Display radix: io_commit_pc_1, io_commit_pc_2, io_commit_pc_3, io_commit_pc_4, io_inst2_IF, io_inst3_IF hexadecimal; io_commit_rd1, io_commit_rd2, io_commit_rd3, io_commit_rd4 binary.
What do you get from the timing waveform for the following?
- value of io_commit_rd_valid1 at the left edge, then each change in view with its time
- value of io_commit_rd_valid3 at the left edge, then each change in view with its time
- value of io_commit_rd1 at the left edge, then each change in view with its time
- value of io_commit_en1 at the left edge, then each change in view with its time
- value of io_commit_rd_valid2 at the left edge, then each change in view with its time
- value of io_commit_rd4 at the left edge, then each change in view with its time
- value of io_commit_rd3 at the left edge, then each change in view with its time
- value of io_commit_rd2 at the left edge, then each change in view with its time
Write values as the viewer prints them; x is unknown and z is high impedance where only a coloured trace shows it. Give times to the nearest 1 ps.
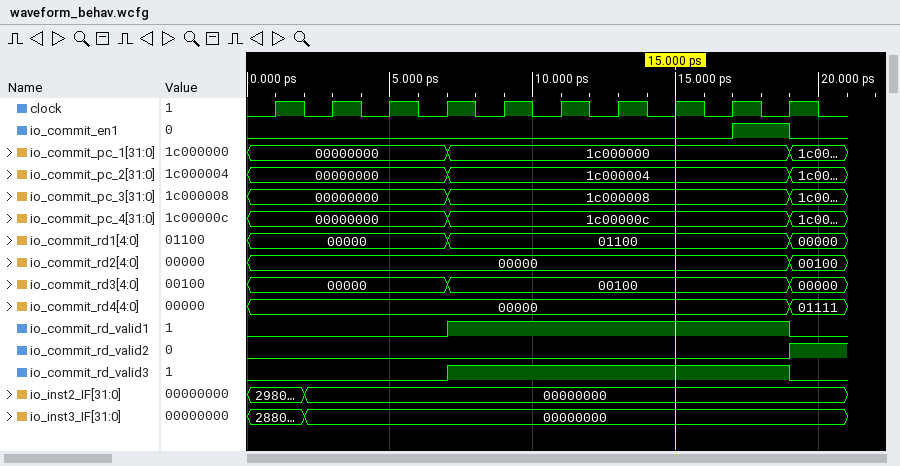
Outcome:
0, 1 at 7 ps, 0 at 19 ps
0, 1 at 7 ps, 0 at 19 ps
00000, 01100 at 7 ps, 00000 at 19 ps
0, 1 at 17 ps, 0 at 19 ps
0, 1 at 19 ps
00000, 01111 at 19 ps
00000, 00100 at 7 ps, 00000 at 19 ps
00000, 00100 at 19 ps
